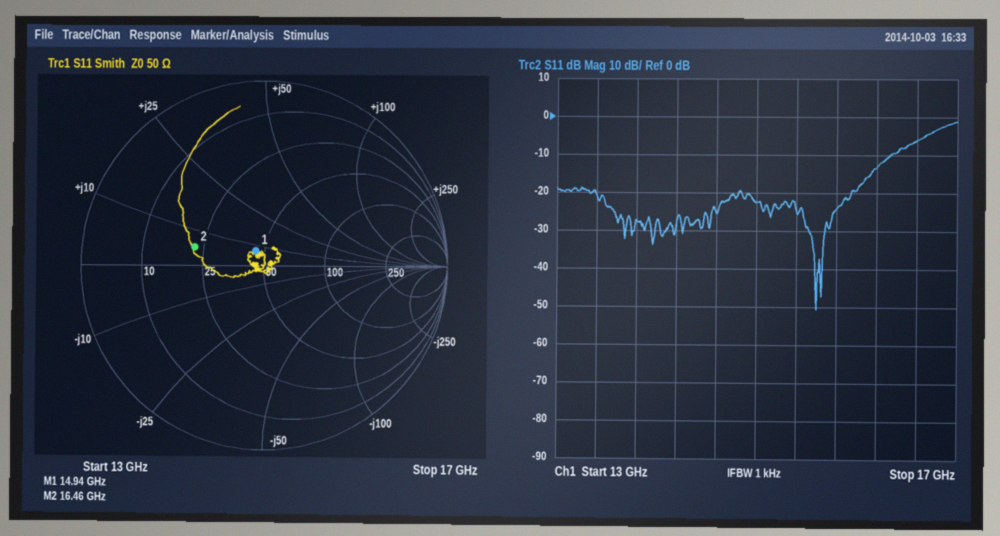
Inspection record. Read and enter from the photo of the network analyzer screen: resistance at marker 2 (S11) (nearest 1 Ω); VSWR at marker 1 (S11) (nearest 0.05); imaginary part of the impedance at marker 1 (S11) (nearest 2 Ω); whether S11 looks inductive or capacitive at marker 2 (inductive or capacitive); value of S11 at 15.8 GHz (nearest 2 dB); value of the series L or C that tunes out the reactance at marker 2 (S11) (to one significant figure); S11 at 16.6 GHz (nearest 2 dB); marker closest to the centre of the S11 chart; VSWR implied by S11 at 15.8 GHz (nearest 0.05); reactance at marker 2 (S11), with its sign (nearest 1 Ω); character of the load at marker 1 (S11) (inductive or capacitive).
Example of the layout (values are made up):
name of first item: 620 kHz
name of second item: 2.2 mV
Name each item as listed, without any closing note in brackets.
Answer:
resistance at marker 2 (S11): 22 Ω
VSWR at marker 1 (S11): 1.20
imaginary part of the impedance at marker 1 (S11): +8 Ω
whether S11 looks inductive or capacitive at marker 2: inductive
value of S11 at 15.8 GHz: -24 dB
value of the series L or C that tunes out the reactance at marker 2 (S11): 2 pF
S11 at 16.6 GHz: -6 dB
marker closest to the centre of the S11 chart: marker 1
VSWR implied by S11 at 15.8 GHz: 1.15
reactance at marker 2 (S11), with its sign: +5 Ω
character of the load at marker 1 (S11): inductive
